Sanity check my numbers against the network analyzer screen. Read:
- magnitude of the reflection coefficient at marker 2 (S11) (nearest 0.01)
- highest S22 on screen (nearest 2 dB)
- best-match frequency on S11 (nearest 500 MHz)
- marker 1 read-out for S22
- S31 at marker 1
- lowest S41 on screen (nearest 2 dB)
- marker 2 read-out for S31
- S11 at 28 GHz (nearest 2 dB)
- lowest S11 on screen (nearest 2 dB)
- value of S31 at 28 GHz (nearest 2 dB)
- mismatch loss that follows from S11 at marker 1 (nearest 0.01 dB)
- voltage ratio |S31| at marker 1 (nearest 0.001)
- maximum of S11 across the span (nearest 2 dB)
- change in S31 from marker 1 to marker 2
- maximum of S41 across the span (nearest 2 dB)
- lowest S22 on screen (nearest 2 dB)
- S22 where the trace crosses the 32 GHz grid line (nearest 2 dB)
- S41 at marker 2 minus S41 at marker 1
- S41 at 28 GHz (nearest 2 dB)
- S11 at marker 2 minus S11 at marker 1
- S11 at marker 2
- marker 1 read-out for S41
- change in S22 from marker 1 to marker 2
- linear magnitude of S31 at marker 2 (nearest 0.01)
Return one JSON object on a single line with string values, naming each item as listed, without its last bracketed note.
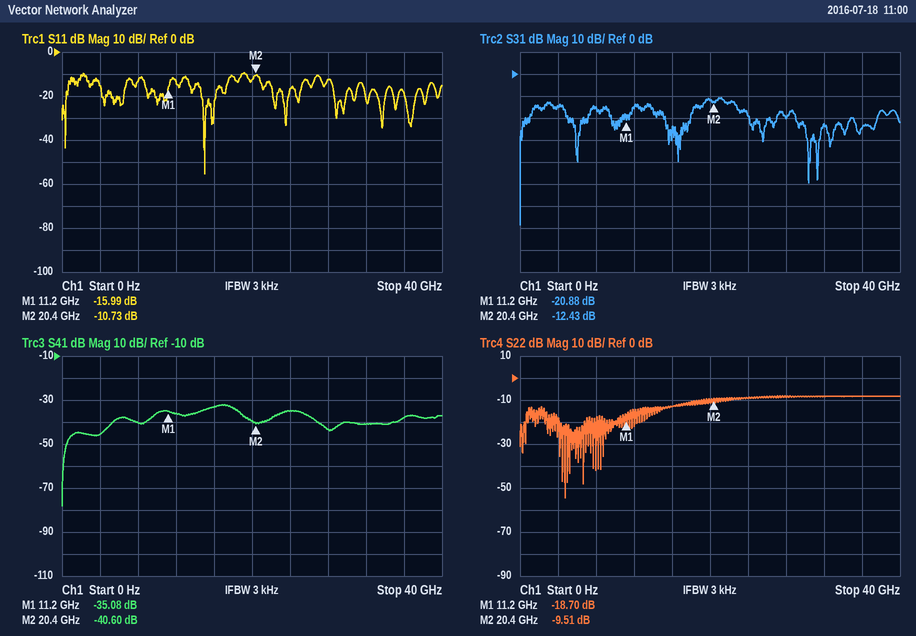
{"magnitude of the reflection coefficient at marker 2 (S11)": "0.29", "highest S22 on screen": "-8 dB", "best-match frequency on S11": "15.0 GHz", "marker 1 read-out for S22": "-18.70 dB", "S31 at marker 1": "-20.88 dB", "lowest S41 on screen": "-78 dB", "marker 2 read-out for S31": "-12.43 dB", "S11 at 28 GHz": "-12 dB", "lowest S11 on screen": "-56 dB", "value of S31 at 28 GHz": "-20 dB", "mismatch loss that follows from S11 at marker 1": "0.11 dB", "voltage ratio |S31| at marker 1": "0.090", "maximum of S11 across the span": "-10 dB", "change in S31 from marker 1 to marker 2": "8.45 dB", "maximum of S41 across the span": "-32 dB", "lowest S22 on screen": "-54 dB", "S22 where the trace crosses the 32 GHz grid line": "-8 dB", "S41 at marker 2 minus S41 at marker 1": "-5.52 dB", "S41 at 28 GHz": "-44 dB", "S11 at marker 2 minus S11 at marker 1": "5.26 dB", "S11 at marker 2": "-10.73 dB", "marker 1 read-out for S41": "-35.08 dB", "change in S22 from marker 1 to marker 2": "9.19 dB", "linear magnitude of S31 at marker 2": "0.24"}
